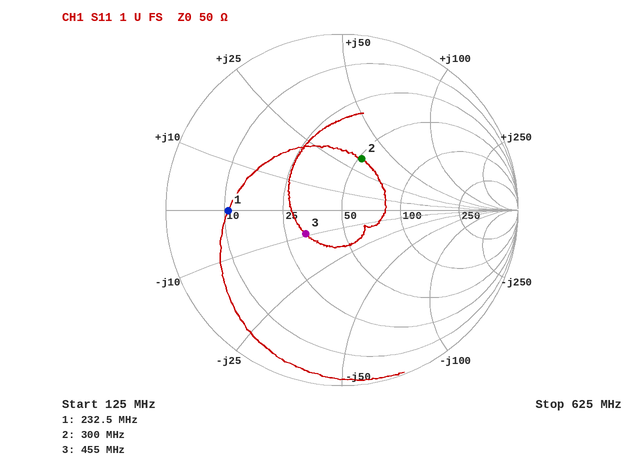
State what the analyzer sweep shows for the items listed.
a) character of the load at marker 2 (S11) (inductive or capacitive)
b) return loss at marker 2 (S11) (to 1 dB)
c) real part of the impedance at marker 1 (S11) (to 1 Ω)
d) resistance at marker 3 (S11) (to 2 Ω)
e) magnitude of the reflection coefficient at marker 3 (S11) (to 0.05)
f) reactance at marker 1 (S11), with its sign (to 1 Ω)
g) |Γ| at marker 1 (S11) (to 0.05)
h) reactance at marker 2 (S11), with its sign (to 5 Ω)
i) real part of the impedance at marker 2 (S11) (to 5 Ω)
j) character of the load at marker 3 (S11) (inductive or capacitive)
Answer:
inductive
10 dB
11 Ω
32 Ω
0.25
0 Ω
0.65
+35 Ω
50 Ω
capacitive
